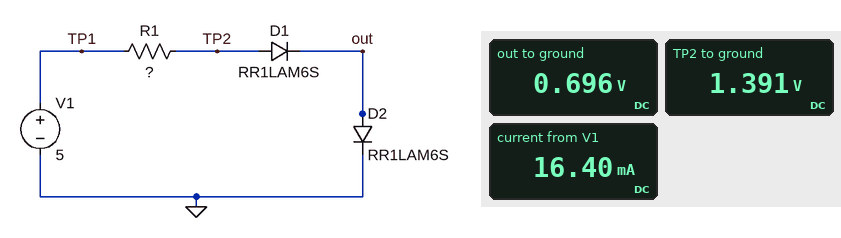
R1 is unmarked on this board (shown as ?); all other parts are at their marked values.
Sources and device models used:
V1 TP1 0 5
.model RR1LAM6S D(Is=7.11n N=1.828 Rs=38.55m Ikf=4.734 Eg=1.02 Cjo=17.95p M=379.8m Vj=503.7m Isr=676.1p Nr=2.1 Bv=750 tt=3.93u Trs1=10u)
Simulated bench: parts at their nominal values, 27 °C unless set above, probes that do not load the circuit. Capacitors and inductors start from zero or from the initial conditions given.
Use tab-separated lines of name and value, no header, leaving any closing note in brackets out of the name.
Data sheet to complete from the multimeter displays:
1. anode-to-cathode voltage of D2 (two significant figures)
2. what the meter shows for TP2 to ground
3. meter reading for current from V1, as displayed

anode-to-cathode voltage of D2	700 mV
what the meter shows for TP2 to ground	1.391 V
meter reading for current from V1, as displayed	16.40 mA
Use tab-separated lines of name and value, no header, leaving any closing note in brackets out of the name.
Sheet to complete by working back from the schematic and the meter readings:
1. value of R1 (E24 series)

value of R1	220 Ω
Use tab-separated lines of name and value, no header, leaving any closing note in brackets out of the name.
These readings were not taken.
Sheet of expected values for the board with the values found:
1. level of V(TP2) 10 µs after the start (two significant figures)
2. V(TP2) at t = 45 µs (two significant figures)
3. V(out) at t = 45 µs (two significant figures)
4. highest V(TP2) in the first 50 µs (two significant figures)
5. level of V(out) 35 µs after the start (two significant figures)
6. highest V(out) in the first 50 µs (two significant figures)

level of V(TP2) 10 µs after the start	1.4 V
V(TP2) at t = 45 µs	1.4 V
V(out) at t = 45 µs	700 mV
highest V(TP2) in the first 50 µs	1.4 V
level of V(out) 35 µs after the start	700 mV
highest V(out) in the first 50 µs	700 mV
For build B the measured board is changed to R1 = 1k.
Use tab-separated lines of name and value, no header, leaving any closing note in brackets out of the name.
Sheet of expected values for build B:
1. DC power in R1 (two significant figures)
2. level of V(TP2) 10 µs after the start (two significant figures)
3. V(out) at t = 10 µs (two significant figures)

DC power in R1	14 mW
level of V(TP2) 10 µs after the start	1.2 V
V(out) at t = 10 µs	620 mV
